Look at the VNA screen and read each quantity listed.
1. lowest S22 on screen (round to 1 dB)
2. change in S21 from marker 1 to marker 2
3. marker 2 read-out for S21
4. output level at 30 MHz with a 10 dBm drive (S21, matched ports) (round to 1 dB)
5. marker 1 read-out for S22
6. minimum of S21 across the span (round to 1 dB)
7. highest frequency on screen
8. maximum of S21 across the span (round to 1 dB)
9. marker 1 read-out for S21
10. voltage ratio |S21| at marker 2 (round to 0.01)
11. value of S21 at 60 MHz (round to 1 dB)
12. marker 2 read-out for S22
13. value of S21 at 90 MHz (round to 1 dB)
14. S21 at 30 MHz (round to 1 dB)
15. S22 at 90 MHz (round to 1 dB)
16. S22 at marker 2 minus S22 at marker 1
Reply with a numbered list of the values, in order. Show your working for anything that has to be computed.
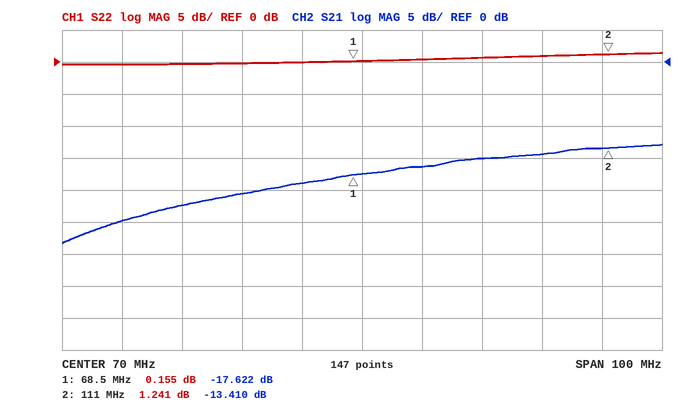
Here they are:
1. 0 dB
2. -13.41 − (-17.622) = 4.212 dB
3. -13.410 dB
4. 10 dBm + (-25 dB) = -15 dBm
5. 0.155 dB
6. -28 dB
7. 120 MHz
8. -13 dB
9. -17.622 dB
10. 10^(-13.41/20) ≈ 0.21
11. -19 dB
12. 1.241 dB
13. -15 dB
14. -25 dB
15. 1 dB
16. 1.241 − (0.155) = 1.086 dB
